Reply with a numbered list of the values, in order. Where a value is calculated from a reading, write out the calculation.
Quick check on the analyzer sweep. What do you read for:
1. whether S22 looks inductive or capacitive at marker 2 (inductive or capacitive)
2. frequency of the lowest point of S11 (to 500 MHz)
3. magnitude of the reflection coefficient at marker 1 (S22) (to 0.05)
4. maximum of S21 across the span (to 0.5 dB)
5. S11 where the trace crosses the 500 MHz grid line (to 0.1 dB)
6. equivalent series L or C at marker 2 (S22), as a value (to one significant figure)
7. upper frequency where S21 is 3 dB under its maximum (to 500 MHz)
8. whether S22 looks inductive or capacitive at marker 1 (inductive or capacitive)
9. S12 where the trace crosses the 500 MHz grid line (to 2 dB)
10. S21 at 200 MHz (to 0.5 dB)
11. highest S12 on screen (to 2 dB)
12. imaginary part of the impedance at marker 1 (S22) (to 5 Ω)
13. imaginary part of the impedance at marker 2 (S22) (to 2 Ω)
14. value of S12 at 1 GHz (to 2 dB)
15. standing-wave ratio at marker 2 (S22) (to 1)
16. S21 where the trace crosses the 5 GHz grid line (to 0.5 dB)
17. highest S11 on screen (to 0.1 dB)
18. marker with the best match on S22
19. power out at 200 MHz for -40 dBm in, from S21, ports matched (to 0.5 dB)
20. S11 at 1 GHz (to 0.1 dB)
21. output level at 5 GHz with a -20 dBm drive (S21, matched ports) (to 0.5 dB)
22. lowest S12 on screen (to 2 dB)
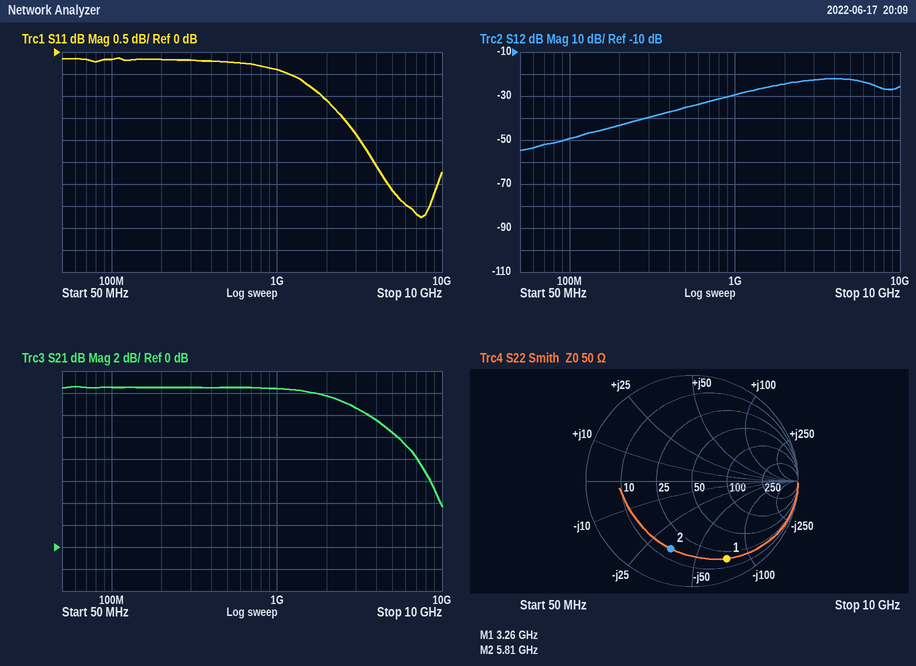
1. capacitive
2. 7.5 GHz
3. 0.80
4. 14.5 dB
5. -0.2 dB
6. C = 1/(2π × 5.81 GHz × 34 Ω) ≈ 806 fF, so 800 fF to one significant figure
7. 4.0 GHz
8. capacitive
9. -36 dB
10. 14.5 dB
11. -22 dB
12. -75 Ω
13. -34 Ω
14. -30 dB
15. 5
16. 10.5 dB
17. -0.1 dB
18. marker 2
19. -40 dBm + (14.5 dB) = -25.5 dBm
20. -0.4 dB
21. -20 dBm + (10.5 dB) = -9.5 dBm
22. -54 dB
